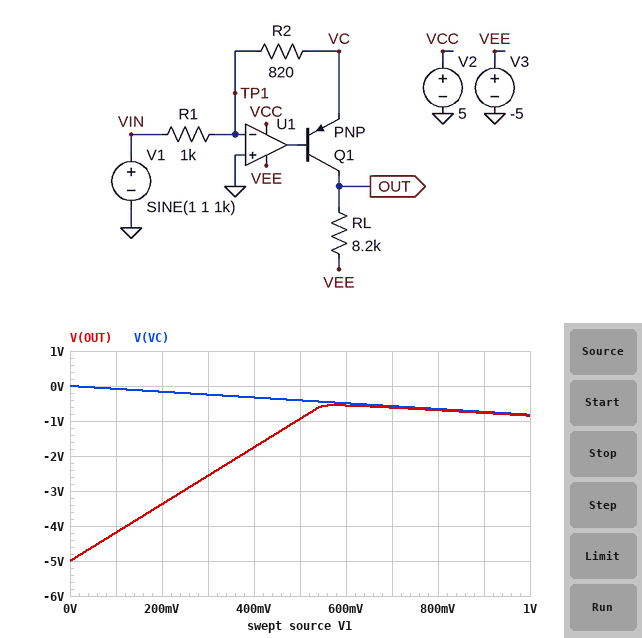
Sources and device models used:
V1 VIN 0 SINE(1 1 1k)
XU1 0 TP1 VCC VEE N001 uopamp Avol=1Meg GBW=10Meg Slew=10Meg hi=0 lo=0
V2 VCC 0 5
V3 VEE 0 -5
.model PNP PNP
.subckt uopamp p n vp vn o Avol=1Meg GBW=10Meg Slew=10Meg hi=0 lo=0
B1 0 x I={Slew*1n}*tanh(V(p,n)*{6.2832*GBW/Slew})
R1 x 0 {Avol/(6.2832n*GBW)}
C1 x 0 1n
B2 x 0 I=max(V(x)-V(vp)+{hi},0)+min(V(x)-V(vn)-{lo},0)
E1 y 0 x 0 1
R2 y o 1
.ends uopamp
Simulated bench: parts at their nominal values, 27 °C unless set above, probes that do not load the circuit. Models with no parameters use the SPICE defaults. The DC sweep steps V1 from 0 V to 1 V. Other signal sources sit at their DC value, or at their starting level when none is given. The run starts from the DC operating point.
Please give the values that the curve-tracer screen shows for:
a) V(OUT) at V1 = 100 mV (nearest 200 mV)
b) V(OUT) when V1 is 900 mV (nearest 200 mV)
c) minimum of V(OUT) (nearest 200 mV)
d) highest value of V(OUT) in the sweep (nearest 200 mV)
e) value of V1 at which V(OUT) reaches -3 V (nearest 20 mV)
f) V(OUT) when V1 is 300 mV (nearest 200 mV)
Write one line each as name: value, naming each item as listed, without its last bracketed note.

V(OUT) at V1 = 100 mV: -4.2 V
V(OUT) when V1 is 900 mV: -800 mV
minimum of V(OUT): -5.0 V
highest value of V(OUT) in the sweep: -600 mV
value of V1 at which V(OUT) reaches -3 V: 240 mV
V(OUT) when V1 is 300 mV: -2.6 V
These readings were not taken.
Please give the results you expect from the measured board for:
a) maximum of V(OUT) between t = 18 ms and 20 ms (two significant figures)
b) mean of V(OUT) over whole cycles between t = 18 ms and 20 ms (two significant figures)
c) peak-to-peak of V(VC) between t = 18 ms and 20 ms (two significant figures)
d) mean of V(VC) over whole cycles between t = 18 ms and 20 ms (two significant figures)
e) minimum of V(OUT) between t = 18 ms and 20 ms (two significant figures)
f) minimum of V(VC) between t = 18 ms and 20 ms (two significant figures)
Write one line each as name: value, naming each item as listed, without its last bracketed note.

maximum of V(OUT) between t = 18 ms and 20 ms: -550 mV
mean of V(OUT) over whole cycles between t = 18 ms and 20 ms: -2.0 V
peak-to-peak of V(VC) between t = 18 ms and 20 ms: 1.6 V
mean of V(VC) over whole cycles between t = 18 ms and 20 ms: -820 mV
minimum of V(OUT) between t = 18 ms and 20 ms: -5.0 V
minimum of V(VC) between t = 18 ms and 20 ms: -1.6 V
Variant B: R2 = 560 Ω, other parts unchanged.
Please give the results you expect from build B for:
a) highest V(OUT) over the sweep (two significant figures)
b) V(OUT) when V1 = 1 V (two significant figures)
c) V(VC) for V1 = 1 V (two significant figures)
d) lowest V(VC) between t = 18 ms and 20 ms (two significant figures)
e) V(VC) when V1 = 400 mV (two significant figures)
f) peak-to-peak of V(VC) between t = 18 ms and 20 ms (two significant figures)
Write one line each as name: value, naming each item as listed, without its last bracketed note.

highest V(OUT) over the sweep: -410 mV
V(OUT) when V1 = 1 V: -590 mV
V(VC) for V1 = 1 V: -560 mV
lowest V(VC) between t = 18 ms and 20 ms: -1.1 V
V(VC) when V1 = 400 mV: -220 mV
peak-to-peak of V(VC) between t = 18 ms and 20 ms: 1.1 V
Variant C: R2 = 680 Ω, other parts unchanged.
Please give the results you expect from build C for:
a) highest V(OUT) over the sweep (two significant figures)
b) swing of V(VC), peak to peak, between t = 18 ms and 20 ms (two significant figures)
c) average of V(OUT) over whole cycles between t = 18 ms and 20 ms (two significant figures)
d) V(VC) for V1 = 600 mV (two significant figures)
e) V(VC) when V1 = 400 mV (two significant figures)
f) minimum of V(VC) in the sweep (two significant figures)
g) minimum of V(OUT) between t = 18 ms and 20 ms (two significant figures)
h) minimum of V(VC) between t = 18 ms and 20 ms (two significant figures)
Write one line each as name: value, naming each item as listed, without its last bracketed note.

highest V(OUT) over the sweep: -480 mV
swing of V(VC), peak to peak, between t = 18 ms and 20 ms: 1.4 V
average of V(OUT) over whole cycles between t = 18 ms and 20 ms: -1.9 V
V(VC) for V1 = 600 mV: -410 mV
V(VC) when V1 = 400 mV: -270 mV
minimum of V(VC) in the sweep: -680 mV
minimum of V(OUT) between t = 18 ms and 20 ms: -5.0 V
minimum of V(VC) between t = 18 ms and 20 ms: -1.4 V
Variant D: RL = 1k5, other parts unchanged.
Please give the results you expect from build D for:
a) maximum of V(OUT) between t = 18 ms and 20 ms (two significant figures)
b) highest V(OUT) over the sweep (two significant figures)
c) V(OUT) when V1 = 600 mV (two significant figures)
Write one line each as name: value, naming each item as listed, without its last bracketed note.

maximum of V(OUT) between t = 18 ms and 20 ms: -2.0 V
highest V(OUT) over the sweep: -3.5 V
V(OUT) when V1 = 600 mV: -4.1 V
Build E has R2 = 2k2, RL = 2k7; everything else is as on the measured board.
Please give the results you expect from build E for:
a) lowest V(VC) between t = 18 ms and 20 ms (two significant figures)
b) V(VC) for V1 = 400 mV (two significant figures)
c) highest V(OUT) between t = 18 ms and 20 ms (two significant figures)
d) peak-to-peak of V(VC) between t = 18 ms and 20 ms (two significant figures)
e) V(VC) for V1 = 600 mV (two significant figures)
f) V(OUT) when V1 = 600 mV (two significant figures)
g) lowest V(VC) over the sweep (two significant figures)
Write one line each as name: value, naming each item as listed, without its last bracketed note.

lowest V(VC) between t = 18 ms and 20 ms: -4.2 V
V(VC) for V1 = 400 mV: -880 mV
highest V(OUT) between t = 18 ms and 20 ms: -2.3 V
peak-to-peak of V(VC) between t = 18 ms and 20 ms: 4.2 V
V(VC) for V1 = 600 mV: -1.3 V
V(OUT) when V1 = 600 mV: -3.4 V
lowest V(VC) over the sweep: -2.2 V
